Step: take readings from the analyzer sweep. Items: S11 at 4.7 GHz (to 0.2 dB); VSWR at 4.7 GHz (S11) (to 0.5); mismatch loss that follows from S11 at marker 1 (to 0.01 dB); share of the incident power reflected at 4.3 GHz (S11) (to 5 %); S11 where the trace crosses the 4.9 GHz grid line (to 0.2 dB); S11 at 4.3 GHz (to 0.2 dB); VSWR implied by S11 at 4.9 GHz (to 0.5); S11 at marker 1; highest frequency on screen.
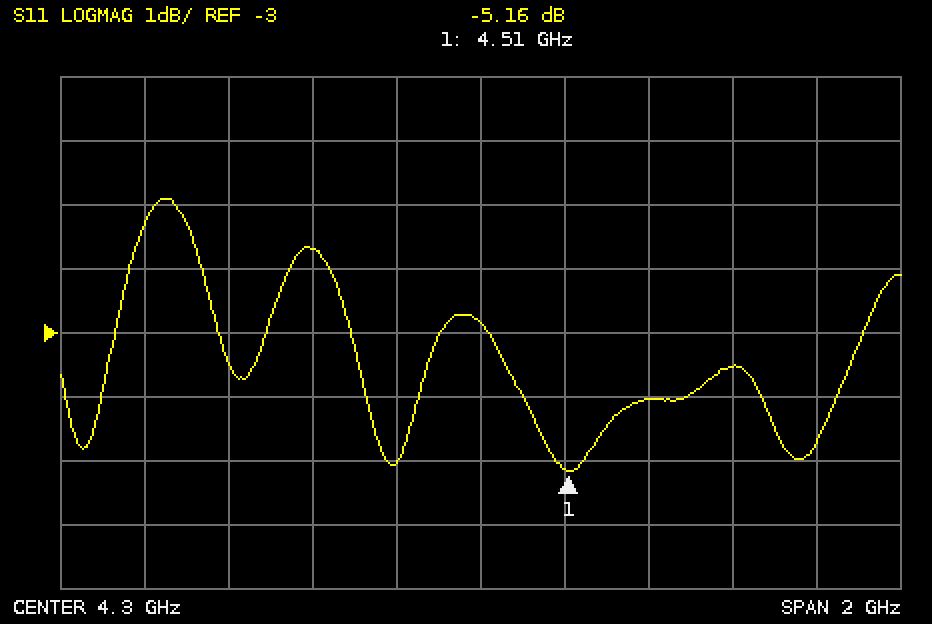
-4.0 dB
4.5
1.58 dB
50 %
-3.6 dB
-2.8 dB
5.0
-5.16 dB
5.3 GHz
